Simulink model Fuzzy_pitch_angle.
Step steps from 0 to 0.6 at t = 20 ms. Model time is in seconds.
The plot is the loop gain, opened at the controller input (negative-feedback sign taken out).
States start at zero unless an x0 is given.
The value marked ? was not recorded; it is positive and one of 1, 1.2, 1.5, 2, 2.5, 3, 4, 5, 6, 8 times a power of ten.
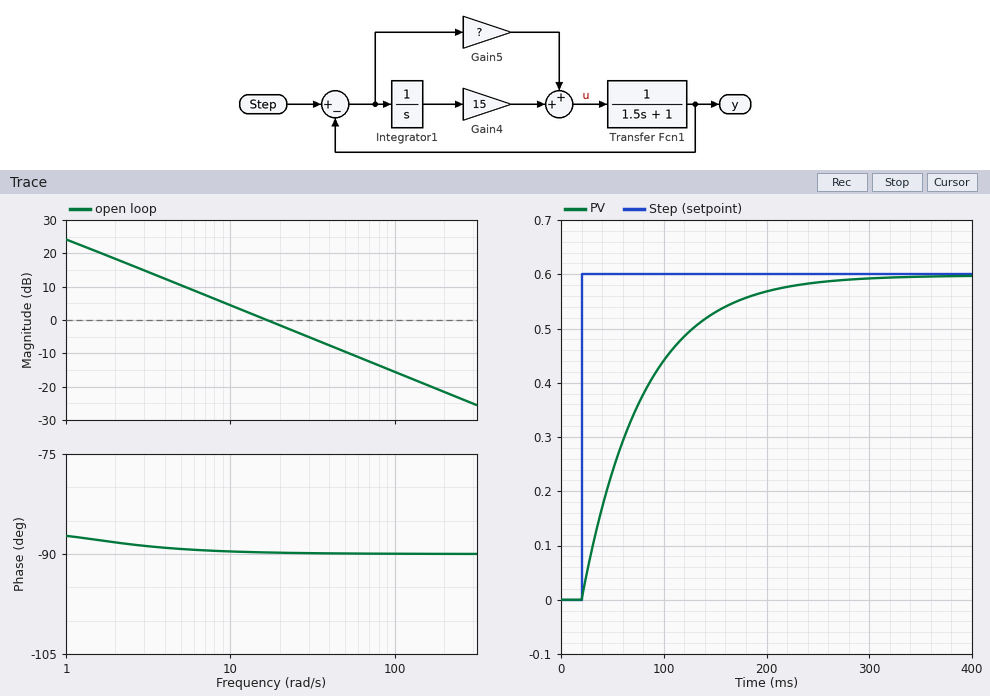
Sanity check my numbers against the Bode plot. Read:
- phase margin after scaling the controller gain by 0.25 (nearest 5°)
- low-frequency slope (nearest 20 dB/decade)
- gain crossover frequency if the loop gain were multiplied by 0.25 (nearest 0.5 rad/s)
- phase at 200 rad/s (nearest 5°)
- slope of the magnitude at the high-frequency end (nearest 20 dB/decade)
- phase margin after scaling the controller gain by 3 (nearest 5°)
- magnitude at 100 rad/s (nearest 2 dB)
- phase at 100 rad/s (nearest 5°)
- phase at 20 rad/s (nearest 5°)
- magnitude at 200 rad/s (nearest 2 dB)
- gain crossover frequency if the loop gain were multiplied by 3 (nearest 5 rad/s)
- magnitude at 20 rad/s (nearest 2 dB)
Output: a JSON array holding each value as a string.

["90°", "-20 dB/decade", "4.0 rad/s", "-90°", "-20 dB/decade", "90°", "-16 dB", "-90°", "-90°", "-22 dB", "50 rad/s", "-2 dB"]
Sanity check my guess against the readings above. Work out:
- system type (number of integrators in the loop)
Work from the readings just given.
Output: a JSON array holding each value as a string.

["1"]
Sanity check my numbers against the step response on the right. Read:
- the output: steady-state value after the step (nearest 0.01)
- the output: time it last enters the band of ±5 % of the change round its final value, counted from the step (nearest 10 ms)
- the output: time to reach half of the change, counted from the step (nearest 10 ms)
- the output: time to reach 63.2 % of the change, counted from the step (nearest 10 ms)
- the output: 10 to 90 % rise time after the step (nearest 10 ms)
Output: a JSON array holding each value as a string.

["0.60", "180 ms", "40 ms", "60 ms", "130 ms"]
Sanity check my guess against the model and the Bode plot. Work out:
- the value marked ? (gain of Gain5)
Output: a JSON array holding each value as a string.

["25"]
